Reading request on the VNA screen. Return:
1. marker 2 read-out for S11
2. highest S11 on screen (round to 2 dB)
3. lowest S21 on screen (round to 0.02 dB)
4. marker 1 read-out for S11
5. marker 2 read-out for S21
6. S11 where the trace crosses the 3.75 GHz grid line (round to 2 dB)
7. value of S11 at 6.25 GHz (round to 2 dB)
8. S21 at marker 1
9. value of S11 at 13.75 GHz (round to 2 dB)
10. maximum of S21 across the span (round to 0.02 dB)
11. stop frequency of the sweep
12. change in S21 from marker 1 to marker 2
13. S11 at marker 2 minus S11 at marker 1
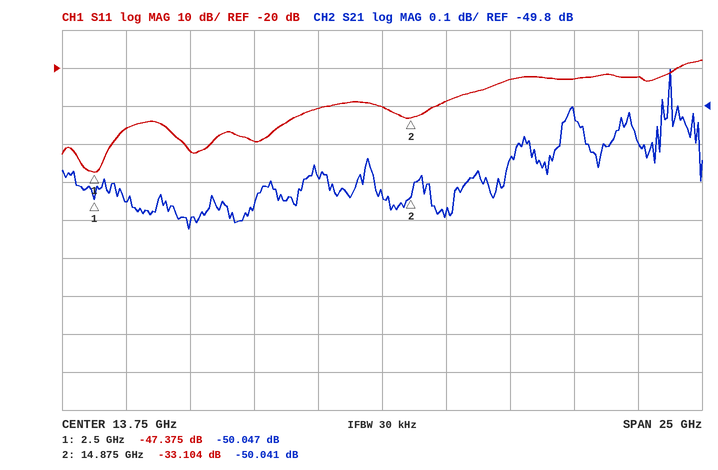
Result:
-33.104 dB
-18 dB
-50.12 dB
-47.375 dB
-50.041 dB
-36 dB
-42 dB
-50.047 dB
-30 dB
-49.70 dB
26.25 GHz
0.006 dB
14.271 dB
